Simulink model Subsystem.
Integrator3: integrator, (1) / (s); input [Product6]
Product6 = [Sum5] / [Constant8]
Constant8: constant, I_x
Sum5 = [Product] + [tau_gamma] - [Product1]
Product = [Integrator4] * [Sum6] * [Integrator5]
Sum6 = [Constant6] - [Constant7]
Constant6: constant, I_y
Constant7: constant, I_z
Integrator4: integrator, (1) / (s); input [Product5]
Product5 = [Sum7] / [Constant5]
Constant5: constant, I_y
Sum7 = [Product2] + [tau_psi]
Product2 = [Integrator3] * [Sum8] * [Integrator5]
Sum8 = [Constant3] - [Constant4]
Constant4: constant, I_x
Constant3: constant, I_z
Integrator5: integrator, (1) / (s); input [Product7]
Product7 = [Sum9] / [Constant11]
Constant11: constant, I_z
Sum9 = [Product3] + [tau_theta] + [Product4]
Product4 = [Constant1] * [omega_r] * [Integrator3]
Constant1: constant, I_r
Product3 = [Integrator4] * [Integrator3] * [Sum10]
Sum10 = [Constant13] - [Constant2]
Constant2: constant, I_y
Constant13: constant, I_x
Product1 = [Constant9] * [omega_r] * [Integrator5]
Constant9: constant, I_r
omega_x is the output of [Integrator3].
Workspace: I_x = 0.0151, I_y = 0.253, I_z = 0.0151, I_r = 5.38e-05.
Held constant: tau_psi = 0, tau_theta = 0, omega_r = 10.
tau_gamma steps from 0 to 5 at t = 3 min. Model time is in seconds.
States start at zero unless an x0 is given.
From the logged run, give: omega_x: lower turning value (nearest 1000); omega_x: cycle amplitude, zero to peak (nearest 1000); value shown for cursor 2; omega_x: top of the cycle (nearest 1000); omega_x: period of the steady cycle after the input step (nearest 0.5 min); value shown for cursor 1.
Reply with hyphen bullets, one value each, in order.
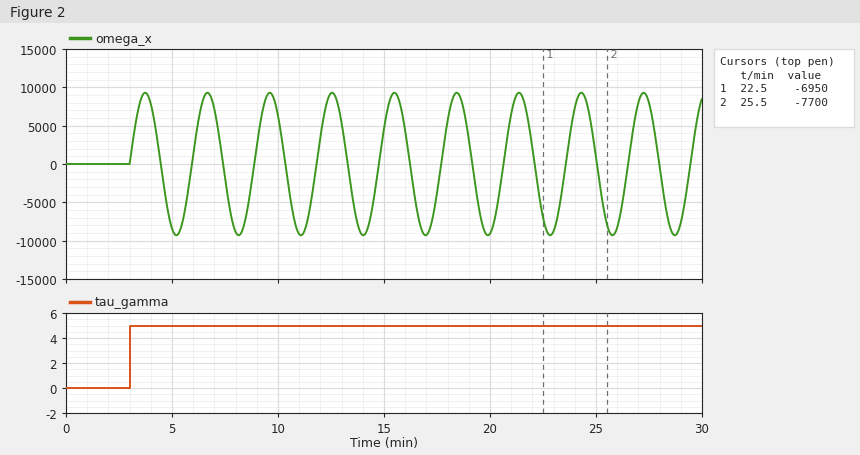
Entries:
- -9000
- 9000
- -7700
- 9000
- 3.0 min
- -6950
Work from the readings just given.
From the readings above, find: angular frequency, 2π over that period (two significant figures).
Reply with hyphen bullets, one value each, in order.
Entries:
- 2.1 rad/min
